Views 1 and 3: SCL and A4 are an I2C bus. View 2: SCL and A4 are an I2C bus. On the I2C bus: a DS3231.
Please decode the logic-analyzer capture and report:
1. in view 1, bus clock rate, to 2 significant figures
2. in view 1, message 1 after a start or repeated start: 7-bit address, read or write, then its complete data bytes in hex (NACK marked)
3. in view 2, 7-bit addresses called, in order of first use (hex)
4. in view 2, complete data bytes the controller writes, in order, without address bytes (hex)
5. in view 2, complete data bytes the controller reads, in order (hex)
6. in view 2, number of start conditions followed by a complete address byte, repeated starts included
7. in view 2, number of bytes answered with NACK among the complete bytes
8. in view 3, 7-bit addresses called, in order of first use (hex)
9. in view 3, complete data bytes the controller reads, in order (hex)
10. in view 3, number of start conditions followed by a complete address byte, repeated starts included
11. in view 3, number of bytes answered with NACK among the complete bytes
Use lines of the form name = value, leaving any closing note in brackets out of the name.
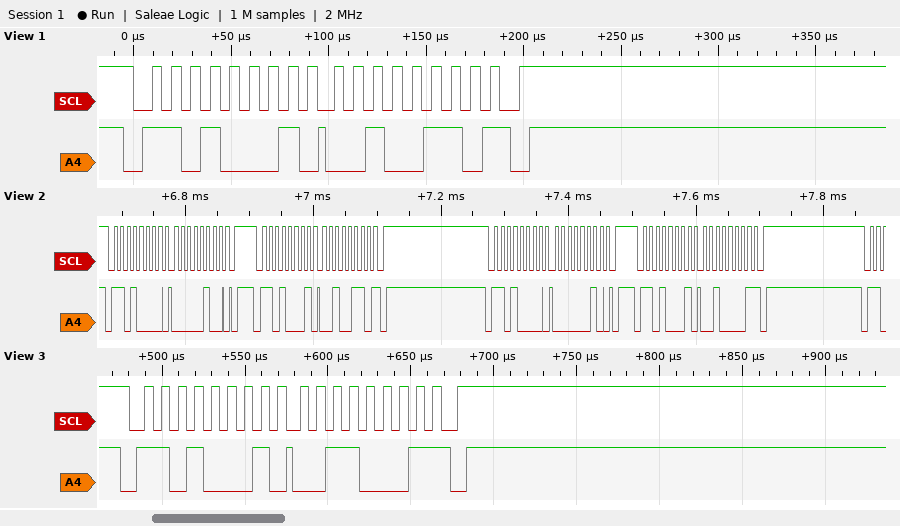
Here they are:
in view 1, bus clock rate, to 2 significant figures = 100 kHz
in view 1, message 1 after a start or repeated start: 7-bit address, read or write, then its complete data bytes in hex = 0x68 read: 26 NACK
in view 2, 7-bit addresses called, in order of first use = 0x68
in view 2, complete data bytes the controller writes, in order, without address bytes = 04 02
in view 2, complete data bytes the controller reads, in order = 26 21
in view 2, number of start conditions followed by a complete address byte, repeated starts included = 4
in view 2, number of bytes answered with NACK among the complete bytes = 2
in view 3, 7-bit addresses called, in order of first use = 0x68
in view 3, complete data bytes the controller reads, in order = 31
in view 3, number of start conditions followed by a complete address byte, repeated starts included = 1
in view 3, number of bytes answered with NACK among the complete bytes = 1
